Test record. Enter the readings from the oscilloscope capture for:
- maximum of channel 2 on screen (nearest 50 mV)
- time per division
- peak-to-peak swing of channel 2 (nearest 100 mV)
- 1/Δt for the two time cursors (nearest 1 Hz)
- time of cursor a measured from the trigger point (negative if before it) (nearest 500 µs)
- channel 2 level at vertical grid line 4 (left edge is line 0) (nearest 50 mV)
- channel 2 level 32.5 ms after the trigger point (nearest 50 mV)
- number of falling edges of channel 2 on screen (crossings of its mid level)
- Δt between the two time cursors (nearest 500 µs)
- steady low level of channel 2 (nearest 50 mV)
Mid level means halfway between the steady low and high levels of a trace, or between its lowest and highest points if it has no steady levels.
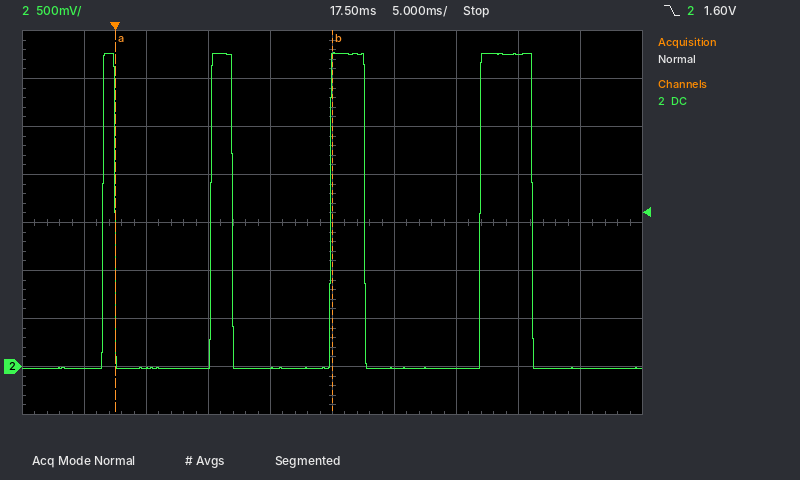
3.25 V
5 ms
3.30 V
57 Hz
0.0 ms
0 mV
3.25 V
4
17.5 ms
0 mV
